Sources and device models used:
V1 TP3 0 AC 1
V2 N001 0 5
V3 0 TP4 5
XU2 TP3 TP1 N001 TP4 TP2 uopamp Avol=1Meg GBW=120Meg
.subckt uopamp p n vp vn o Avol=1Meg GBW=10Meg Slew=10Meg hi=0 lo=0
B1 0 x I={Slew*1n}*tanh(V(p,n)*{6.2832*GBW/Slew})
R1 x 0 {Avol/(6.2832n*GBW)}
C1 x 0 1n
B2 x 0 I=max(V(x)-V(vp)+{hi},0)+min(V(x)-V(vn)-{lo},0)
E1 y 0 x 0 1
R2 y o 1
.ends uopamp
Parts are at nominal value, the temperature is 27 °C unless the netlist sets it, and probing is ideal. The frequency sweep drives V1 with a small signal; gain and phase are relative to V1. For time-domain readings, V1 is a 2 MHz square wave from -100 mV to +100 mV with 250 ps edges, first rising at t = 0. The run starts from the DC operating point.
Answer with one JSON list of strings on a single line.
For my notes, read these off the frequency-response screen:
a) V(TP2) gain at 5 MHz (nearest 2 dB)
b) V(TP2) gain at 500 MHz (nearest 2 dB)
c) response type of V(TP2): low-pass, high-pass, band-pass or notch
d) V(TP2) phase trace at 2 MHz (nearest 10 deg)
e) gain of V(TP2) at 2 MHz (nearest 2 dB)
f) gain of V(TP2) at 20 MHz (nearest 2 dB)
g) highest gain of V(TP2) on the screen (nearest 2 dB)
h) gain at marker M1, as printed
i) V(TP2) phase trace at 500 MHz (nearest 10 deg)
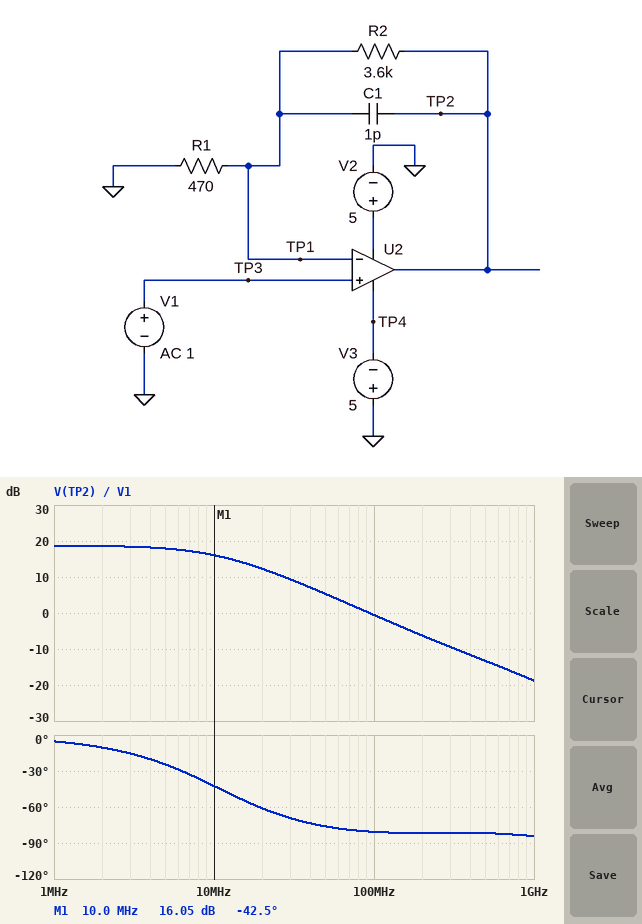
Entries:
["18 dB", "-14 dB", "low-pass", "-10 deg", "18 dB", "12 dB", "18 dB", "16.05 dB", "-80 deg"]
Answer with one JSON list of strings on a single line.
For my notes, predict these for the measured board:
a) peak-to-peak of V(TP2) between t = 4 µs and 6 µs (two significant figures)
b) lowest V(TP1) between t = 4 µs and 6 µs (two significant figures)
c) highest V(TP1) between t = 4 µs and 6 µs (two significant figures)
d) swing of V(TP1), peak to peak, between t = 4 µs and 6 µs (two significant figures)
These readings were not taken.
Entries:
["1.7 V", "-100 mV", "100 mV", "200 mV"]
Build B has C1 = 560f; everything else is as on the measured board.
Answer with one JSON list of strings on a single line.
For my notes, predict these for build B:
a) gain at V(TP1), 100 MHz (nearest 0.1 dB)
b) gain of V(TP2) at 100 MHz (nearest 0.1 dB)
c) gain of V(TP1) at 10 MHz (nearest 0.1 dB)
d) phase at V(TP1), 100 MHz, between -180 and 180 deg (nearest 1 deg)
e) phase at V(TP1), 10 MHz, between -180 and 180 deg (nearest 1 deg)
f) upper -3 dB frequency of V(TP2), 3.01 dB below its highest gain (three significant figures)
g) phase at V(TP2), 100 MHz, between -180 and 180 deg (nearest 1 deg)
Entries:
["-14.4 dB", "0.3 dB", "-2.2 dB", "-39 deg", "-33 deg", "12.0 MHz", "-82 deg"]
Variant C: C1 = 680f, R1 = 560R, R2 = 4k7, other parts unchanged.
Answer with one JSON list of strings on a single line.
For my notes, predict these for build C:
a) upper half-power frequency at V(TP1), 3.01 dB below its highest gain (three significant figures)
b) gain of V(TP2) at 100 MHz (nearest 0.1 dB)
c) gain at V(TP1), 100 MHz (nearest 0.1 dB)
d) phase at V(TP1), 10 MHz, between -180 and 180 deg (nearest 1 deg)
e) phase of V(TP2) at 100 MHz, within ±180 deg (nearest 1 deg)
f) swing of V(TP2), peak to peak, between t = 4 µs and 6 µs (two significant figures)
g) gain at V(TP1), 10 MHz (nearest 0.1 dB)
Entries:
["10.8 MHz", "-0.2 dB", "-12.9 dB", "-34 deg", "-82 deg", "1.9 V", "-2.7 dB"]
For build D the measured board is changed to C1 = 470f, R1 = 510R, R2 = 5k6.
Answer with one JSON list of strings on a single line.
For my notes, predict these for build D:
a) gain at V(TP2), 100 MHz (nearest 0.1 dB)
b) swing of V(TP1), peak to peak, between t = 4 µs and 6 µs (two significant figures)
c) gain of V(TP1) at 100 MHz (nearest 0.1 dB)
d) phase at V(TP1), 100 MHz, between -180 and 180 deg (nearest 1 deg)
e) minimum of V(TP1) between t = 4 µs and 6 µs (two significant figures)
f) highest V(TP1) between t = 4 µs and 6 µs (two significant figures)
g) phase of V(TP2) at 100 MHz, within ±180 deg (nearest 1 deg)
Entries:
["0.3 dB", "190 mV", "-15.6 dB", "-33 deg", "-97 mV", "97 mV", "-84 deg"]
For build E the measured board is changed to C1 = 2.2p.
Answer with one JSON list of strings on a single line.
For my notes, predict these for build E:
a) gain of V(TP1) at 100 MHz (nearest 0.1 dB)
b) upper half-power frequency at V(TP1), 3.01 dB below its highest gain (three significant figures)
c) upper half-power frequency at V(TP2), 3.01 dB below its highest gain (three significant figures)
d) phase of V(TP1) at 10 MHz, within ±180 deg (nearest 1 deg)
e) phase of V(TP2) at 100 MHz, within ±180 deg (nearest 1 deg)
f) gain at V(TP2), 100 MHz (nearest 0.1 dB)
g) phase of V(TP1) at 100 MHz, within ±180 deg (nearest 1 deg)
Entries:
["-7.9 dB", "10.5 MHz", "8.46 MHz", "-25 deg", "-75 deg", "-2.0 dB", "-26 deg"]
